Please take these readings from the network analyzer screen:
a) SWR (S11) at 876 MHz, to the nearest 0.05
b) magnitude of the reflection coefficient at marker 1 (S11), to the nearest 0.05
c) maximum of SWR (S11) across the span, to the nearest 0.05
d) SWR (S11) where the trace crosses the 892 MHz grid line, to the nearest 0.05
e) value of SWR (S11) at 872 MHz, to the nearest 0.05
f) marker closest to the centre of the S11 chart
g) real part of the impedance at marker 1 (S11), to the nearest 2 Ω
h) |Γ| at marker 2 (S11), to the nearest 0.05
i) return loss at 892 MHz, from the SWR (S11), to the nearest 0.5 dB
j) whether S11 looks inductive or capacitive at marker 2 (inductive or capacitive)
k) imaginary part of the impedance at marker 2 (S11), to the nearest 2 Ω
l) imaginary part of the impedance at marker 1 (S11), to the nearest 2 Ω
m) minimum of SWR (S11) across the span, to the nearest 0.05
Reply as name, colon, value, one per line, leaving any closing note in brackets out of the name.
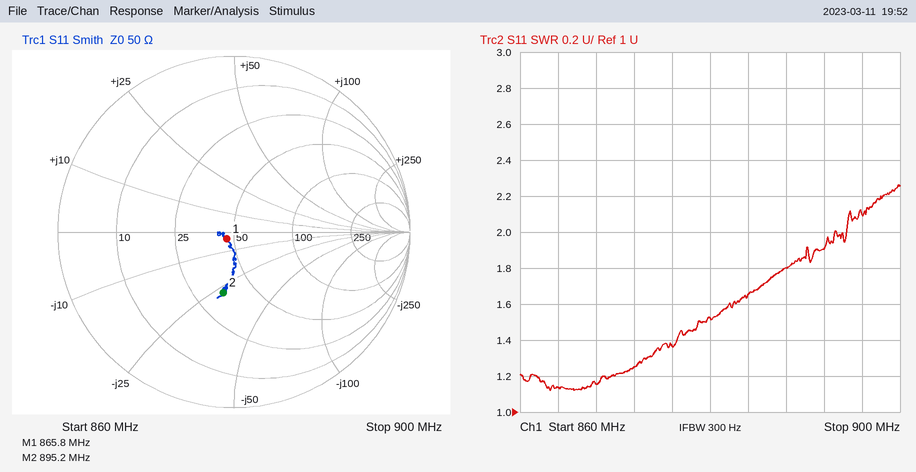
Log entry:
SWR (S11) at 876 MHz, to the nearest 0.05: 1.35
magnitude of the reflection coefficient at marker 1 (S11), to the nearest 0.05: 0.05
maximum of SWR (S11) across the span, to the nearest 0.05: 2.25
SWR (S11) where the trace crosses the 892 MHz grid line, to the nearest 0.05: 1.90
value of SWR (S11) at 872 MHz, to the nearest 0.05: 1.25
marker closest to the centre of the S11 chart: marker 1
real part of the impedance at marker 1 (S11), to the nearest 2 Ω: 46 Ω
|Γ| at marker 2 (S11), to the nearest 0.05: 0.35
return loss at 892 MHz, from the SWR (S11), to the nearest 0.5 dB: 10.0 dB
whether S11 looks inductive or capacitive at marker 2: capacitive
imaginary part of the impedance at marker 2 (S11), to the nearest 2 Ω: -28 Ω
imaginary part of the impedance at marker 1 (S11), to the nearest 2 Ω: -4 Ω
minimum of SWR (S11) across the span, to the nearest 0.05: 1.10
